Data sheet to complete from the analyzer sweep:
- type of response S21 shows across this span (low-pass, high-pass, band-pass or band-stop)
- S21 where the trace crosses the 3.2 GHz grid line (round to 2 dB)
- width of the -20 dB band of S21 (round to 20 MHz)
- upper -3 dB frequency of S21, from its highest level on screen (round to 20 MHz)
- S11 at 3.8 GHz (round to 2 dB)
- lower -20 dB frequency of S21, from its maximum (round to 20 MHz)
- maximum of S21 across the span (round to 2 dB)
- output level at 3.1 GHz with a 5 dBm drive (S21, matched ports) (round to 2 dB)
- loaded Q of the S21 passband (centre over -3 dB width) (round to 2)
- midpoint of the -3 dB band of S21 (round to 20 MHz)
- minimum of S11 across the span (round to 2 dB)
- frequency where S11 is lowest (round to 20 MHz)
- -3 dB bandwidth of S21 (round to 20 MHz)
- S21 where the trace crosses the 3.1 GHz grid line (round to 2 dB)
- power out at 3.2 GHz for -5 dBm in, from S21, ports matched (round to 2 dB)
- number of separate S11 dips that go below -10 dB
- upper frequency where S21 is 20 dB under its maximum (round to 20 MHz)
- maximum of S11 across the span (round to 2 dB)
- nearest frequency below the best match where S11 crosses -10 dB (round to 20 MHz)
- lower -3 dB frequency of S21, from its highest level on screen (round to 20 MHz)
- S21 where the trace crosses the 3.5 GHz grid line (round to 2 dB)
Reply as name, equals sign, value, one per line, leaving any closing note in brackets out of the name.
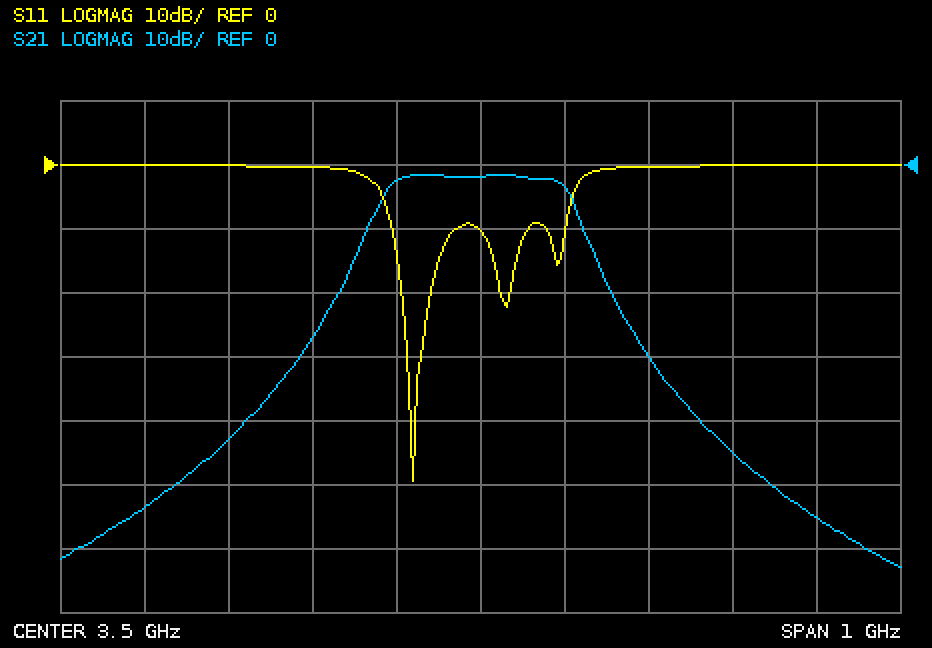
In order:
type of response S21 shows across this span = band-pass
S21 where the trace crosses the 3.2 GHz grid line = -42 dB
width of the -20 dB band of S21 = 340 MHz
upper -3 dB frequency of S21, from its highest level on screen = 3.60 GHz
S11 at 3.8 GHz = 0 dB
lower -20 dB frequency of S21, from its maximum = 3.32 GHz
maximum of S21 across the span = -2 dB
output level at 3.1 GHz with a 5 dBm drive (S21, matched ports) = -48 dBm
loaded Q of the S21 passband (centre over -3 dB width) = 16
midpoint of the -3 dB band of S21 = 3.50 GHz
minimum of S11 across the span = -50 dB
frequency where S11 is lowest = 3.42 GHz
-3 dB bandwidth of S21 = 220 MHz
S21 where the trace crosses the 3.1 GHz grid line = -54 dB
power out at 3.2 GHz for -5 dBm in, from S21, ports matched = -48 dBm
number of separate S11 dips that go below -10 dB = 3
upper frequency where S21 is 20 dB under its maximum = 3.66 GHz
maximum of S11 across the span = 0 dB
nearest frequency below the best match where S11 crosses -10 dB = 3.40 GHz
lower -3 dB frequency of S21, from its highest level on screen = 3.38 GHz
S21 where the trace crosses the 3.5 GHz grid line = -2 dB
